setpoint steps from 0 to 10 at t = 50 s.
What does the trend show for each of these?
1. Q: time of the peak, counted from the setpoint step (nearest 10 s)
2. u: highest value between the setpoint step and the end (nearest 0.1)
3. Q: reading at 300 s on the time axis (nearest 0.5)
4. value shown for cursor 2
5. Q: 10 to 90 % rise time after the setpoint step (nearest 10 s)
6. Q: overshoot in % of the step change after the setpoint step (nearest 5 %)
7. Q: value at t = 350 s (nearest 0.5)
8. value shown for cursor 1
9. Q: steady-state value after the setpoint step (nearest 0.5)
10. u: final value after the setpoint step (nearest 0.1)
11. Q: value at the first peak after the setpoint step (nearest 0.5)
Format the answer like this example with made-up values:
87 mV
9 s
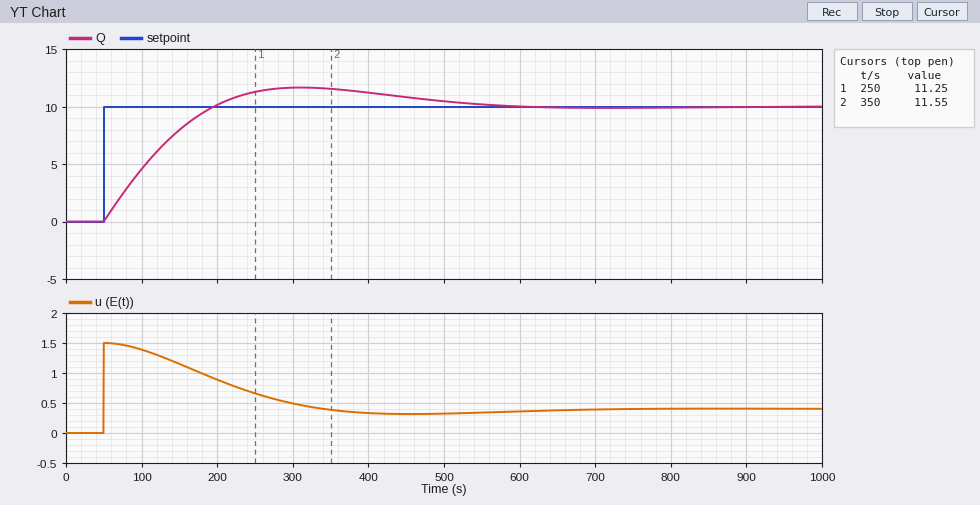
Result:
260 s
1.5
11.5
11.55
110 s
15 %
11.5
11.25
10.0
0.4
11.5
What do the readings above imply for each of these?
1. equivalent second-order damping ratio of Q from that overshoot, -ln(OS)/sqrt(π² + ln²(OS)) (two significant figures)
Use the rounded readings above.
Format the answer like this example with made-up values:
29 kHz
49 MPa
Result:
0.52
